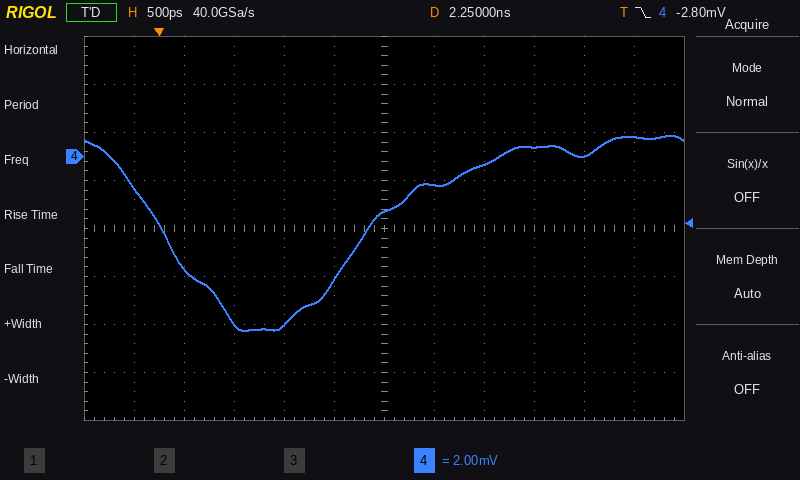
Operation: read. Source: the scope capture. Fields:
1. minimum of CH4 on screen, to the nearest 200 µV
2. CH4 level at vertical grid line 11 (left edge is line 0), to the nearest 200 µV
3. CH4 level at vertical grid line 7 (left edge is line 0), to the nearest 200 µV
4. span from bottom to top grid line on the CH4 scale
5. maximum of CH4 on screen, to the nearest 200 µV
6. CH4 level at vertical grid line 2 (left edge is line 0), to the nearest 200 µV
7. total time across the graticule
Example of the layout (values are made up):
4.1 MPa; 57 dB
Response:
-7.2 mV; 800 µV; -1.2 mV; 16 mV; 800 µV; -4.6 mV; 6 ns
